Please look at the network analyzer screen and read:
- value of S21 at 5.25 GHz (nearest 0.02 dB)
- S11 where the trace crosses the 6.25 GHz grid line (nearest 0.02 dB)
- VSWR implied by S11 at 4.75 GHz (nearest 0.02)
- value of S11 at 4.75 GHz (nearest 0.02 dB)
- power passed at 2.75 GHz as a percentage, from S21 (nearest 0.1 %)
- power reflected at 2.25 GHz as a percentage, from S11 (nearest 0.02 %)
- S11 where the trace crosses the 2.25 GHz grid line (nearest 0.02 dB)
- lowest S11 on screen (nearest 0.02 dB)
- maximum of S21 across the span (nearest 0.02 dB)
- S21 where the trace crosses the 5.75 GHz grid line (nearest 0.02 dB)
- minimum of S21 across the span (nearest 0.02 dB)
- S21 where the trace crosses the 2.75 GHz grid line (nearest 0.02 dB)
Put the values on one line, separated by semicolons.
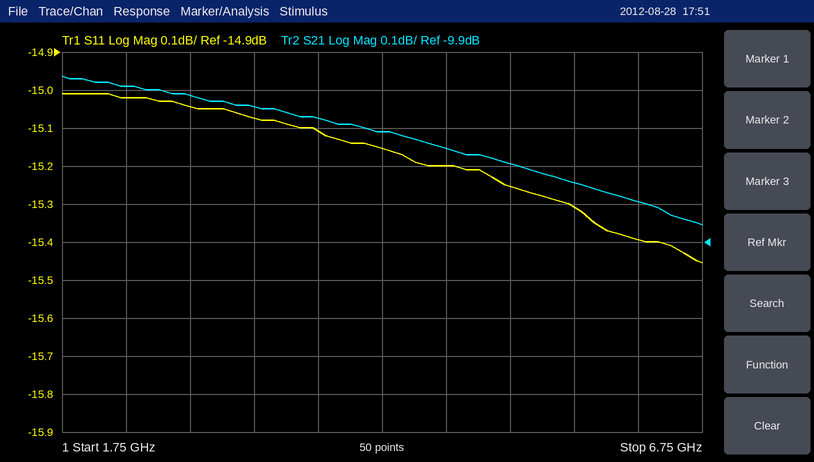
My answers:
-9.70 dB; -15.40 dB; 1.42; -15.20 dB; 11.2 %; 3.14 %; -15.02 dB; -15.46 dB; -9.46 dB; -9.74 dB; -9.86 dB; -9.52 dB
